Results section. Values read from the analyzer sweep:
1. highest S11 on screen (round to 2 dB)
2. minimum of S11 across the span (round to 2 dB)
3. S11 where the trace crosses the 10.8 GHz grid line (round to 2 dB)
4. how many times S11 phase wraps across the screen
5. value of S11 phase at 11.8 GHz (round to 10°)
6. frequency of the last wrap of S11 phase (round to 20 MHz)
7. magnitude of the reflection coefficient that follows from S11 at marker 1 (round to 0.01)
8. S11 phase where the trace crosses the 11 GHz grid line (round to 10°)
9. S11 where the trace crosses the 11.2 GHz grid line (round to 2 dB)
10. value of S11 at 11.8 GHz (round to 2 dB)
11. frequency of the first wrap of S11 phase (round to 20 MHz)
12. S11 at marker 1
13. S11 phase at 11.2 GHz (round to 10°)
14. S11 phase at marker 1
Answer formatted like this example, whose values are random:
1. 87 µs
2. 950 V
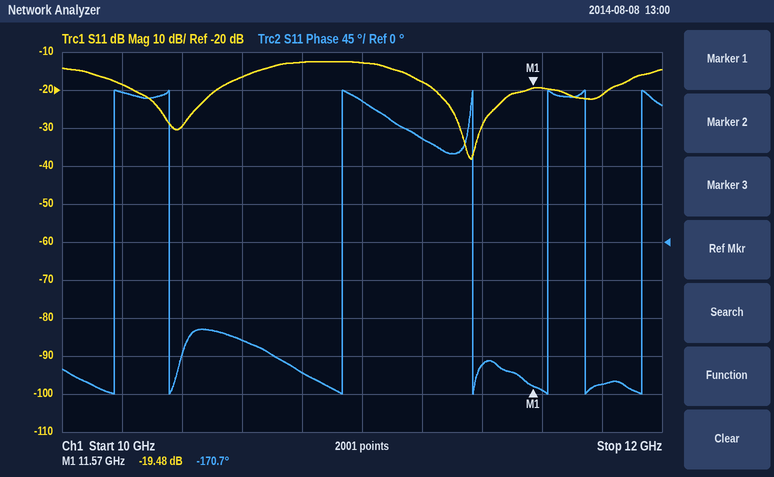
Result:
1. -12 dB
2. -38 dB
3. -12 dB
4. 7
5. -170°
6. 11.94 GHz
7. 0.11
8. 170°
9. -18 dB
10. -22 dB
11. 10.18 GHz
12. -19.48 dB
13. 120°
14. -170.7°
